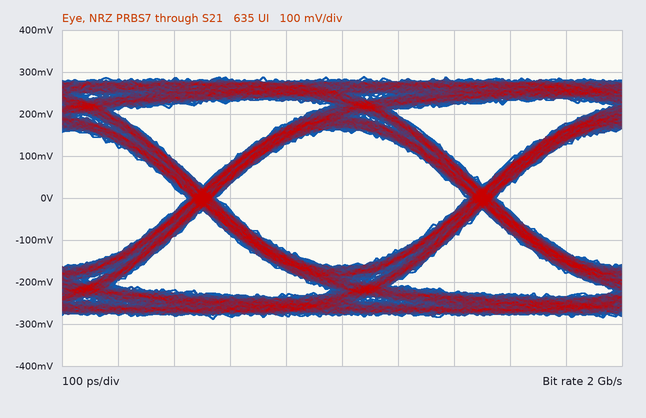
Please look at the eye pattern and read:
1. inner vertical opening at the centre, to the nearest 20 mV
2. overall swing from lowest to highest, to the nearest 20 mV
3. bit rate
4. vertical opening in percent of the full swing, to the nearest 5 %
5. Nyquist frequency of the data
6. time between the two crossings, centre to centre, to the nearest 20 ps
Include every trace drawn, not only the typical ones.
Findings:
320 mV
580 mV
2 Gb/s
55 %
1 GHz
500 ps
